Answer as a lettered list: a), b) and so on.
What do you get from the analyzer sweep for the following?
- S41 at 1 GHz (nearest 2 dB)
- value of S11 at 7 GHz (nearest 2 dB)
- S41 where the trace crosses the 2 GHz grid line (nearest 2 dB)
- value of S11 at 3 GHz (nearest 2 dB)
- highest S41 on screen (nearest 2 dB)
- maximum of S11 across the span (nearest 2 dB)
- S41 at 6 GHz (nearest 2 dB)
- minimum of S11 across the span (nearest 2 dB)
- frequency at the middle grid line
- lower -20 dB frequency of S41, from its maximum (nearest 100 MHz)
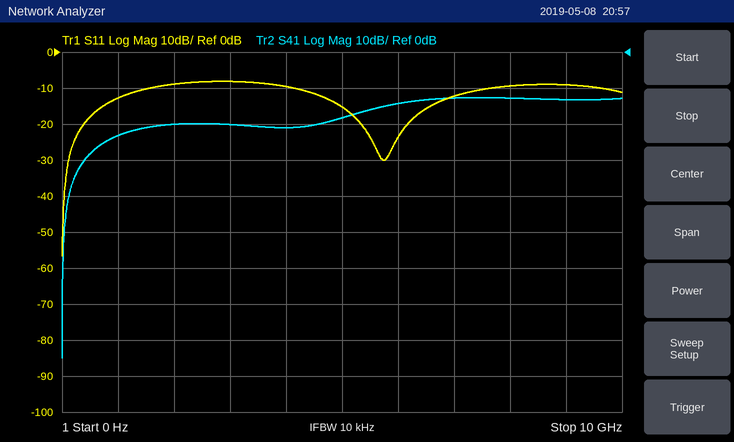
a) -24 dB
b) -12 dB
c) -20 dB
d) -8 dB
e) -12 dB
f) -8 dB
g) -14 dB
h) -56 dB
i) 5 GHz
j) 300 MHz
